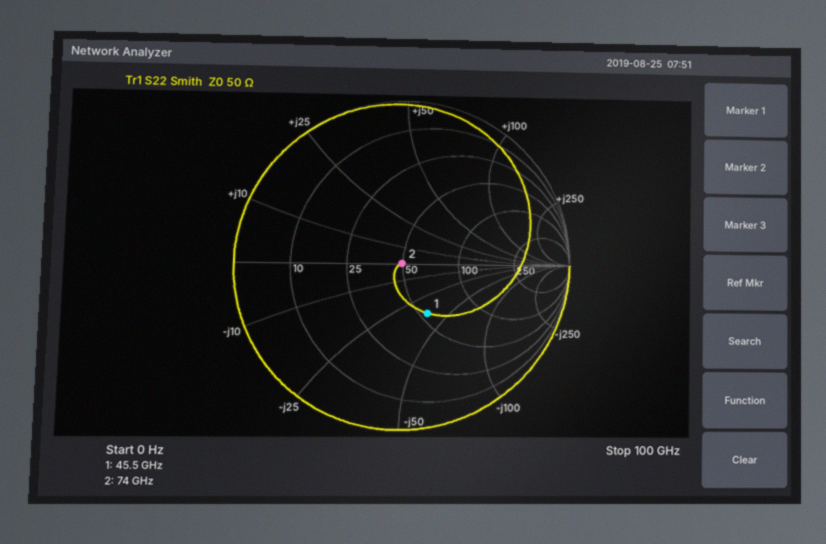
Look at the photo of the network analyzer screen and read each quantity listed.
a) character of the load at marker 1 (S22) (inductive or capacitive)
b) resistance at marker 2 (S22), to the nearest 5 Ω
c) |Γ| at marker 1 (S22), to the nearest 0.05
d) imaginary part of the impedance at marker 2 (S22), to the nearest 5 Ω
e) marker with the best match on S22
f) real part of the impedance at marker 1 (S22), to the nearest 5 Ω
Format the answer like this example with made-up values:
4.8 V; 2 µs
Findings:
capacitive; 50 Ω; 0.35; 0 Ω; marker 2; 55 Ω
